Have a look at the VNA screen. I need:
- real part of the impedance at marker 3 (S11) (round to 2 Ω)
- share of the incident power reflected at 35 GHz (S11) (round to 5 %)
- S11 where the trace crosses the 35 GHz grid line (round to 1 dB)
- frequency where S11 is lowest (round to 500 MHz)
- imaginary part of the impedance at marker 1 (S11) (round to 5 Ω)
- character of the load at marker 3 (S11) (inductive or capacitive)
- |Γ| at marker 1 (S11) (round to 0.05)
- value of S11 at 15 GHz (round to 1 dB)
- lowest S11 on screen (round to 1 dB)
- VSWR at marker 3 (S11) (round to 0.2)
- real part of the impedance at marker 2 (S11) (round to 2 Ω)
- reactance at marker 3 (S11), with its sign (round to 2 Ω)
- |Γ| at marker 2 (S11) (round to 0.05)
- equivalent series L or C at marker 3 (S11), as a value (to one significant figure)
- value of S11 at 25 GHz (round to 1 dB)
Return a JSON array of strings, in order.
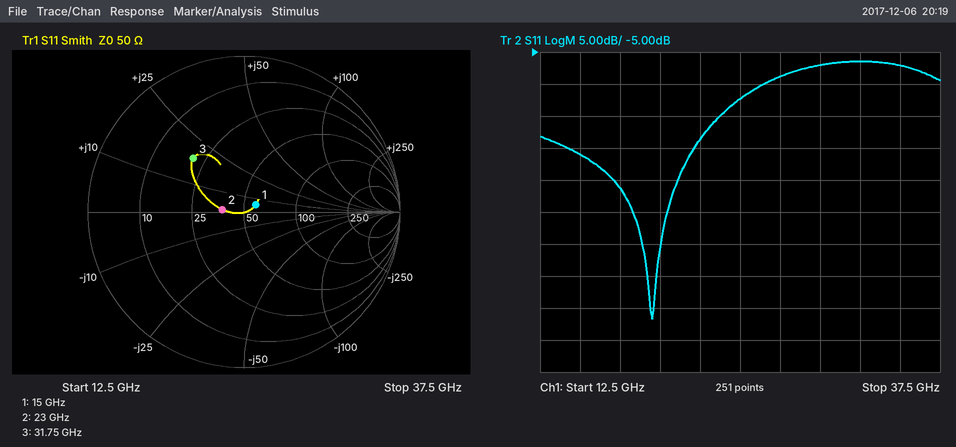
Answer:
["20 Ω", "20 %", "-7 dB", "19.5 GHz", "+5 Ω", "inductive", "0.10", "-21 dB", "-47 dB", "2.8", "38 Ω", "+18 Ω", "0.15", "90 pH", "-12 dB"]
